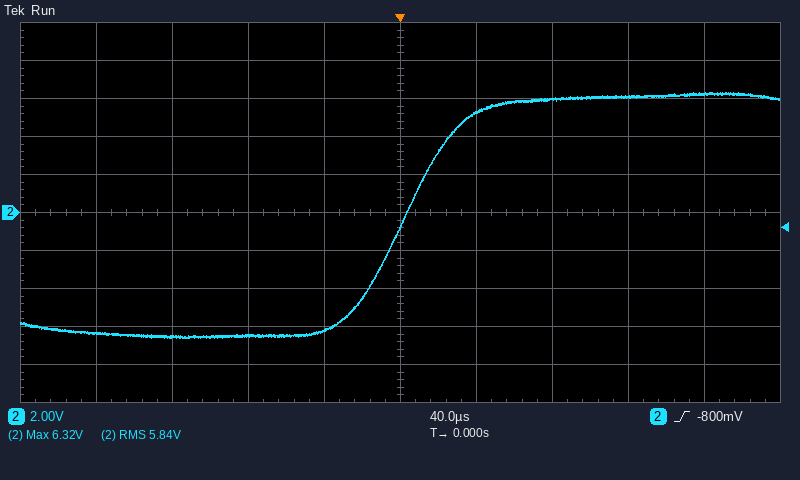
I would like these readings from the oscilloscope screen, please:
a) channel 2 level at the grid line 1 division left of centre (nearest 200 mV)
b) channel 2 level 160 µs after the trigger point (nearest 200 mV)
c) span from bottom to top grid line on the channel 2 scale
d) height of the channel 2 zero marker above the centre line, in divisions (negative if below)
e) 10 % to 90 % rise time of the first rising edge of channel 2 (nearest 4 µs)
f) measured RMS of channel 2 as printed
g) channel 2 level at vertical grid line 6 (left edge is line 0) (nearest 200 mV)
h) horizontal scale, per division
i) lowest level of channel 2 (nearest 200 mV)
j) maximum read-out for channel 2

-6.2 V
6.2 V
20 V
0.0 div
60 µs
5.84 V
5.2 V
40 µs
-6.6 V
6.32 V
